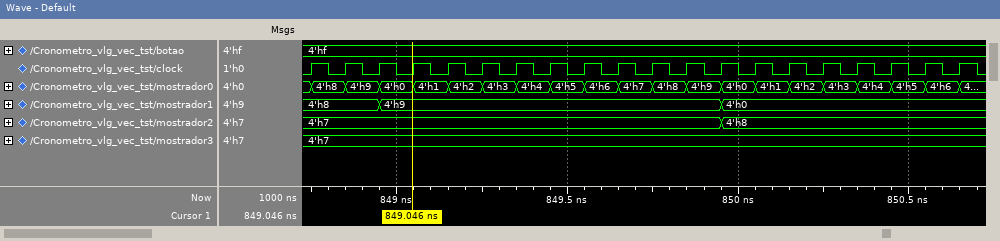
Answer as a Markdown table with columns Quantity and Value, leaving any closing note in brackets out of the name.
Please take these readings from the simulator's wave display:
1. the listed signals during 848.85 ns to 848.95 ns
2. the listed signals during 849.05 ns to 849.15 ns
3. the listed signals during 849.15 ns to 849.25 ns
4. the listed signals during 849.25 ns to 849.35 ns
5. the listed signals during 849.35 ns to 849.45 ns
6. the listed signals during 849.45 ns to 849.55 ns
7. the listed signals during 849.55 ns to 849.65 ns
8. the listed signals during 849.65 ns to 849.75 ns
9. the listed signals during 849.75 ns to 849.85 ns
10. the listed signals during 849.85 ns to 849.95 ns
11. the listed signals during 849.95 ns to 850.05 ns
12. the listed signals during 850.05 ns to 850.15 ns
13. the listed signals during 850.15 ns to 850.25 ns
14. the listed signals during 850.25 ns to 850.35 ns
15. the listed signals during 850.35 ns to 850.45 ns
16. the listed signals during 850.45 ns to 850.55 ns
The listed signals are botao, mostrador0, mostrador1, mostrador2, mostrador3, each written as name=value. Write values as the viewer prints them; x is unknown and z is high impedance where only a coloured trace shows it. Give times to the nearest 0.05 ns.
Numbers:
| Quantity | Value |
|---|---|
| the listed signals during 848.85 ns to 848.95 ns | botao=4'hf, mostrador0=4'h9, mostrador1=4'h8, mostrador2=4'h7, mostrador3=4'h7 |
| the listed signals during 849.05 ns to 849.15 ns | botao=4'hf, mostrador0=4'h1, mostrador1=4'h9, mostrador2=4'h7, mostrador3=4'h7 |
| the listed signals during 849.15 ns to 849.25 ns | botao=4'hf, mostrador0=4'h2, mostrador1=4'h9, mostrador2=4'h7, mostrador3=4'h7 |
| the listed signals during 849.25 ns to 849.35 ns | botao=4'hf, mostrador0=4'h3, mostrador1=4'h9, mostrador2=4'h7, mostrador3=4'h7 |
| the listed signals during 849.35 ns to 849.45 ns | botao=4'hf, mostrador0=4'h4, mostrador1=4'h9, mostrador2=4'h7, mostrador3=4'h7 |
| the listed signals during 849.45 ns to 849.55 ns | botao=4'hf, mostrador0=4'h5, mostrador1=4'h9, mostrador2=4'h7, mostrador3=4'h7 |
| the listed signals during 849.55 ns to 849.65 ns | botao=4'hf, mostrador0=4'h6, mostrador1=4'h9, mostrador2=4'h7, mostrador3=4'h7 |
| the listed signals during 849.65 ns to 849.75 ns | botao=4'hf, mostrador0=4'h7, mostrador1=4'h9, mostrador2=4'h7, mostrador3=4'h7 |
| the listed signals during 849.75 ns to 849.85 ns | botao=4'hf, mostrador0=4'h8, mostrador1=4'h9, mostrador2=4'h7, mostrador3=4'h7 |
| the listed signals during 849.85 ns to 849.95 ns | botao=4'hf, mostrador0=4'h9, mostrador1=4'h9, mostrador2=4'h7, mostrador3=4'h7 |
| the listed signals during 849.95 ns to 850.05 ns | botao=4'hf, mostrador0=4'h0, mostrador1=4'h0, mostrador2=4'h8, mostrador3=4'h7 |
| the listed signals during 850.05 ns to 850.15 ns | botao=4'hf, mostrador0=4'h1, mostrador1=4'h0, mostrador2=4'h8, mostrador3=4'h7 |
| the listed signals during 850.15 ns to 850.25 ns | botao=4'hf, mostrador0=4'h2, mostrador1=4'h0, mostrador2=4'h8, mostrador3=4'h7 |
| the listed signals during 850.25 ns to 850.35 ns | botao=4'hf, mostrador0=4'h3, mostrador1=4'h0, mostrador2=4'h8, mostrador3=4'h7 |
| the listed signals during 850.35 ns to 850.45 ns | botao=4'hf, mostrador0=4'h4, mostrador1=4'h0, mostrador2=4'h8, mostrador3=4'h7 |
| the listed signals during 850.45 ns to 850.55 ns | botao=4'hf, mostrador0=4'h5, mostrador1=4'h0, mostrador2=4'h8, mostrador3=4'h7 |
